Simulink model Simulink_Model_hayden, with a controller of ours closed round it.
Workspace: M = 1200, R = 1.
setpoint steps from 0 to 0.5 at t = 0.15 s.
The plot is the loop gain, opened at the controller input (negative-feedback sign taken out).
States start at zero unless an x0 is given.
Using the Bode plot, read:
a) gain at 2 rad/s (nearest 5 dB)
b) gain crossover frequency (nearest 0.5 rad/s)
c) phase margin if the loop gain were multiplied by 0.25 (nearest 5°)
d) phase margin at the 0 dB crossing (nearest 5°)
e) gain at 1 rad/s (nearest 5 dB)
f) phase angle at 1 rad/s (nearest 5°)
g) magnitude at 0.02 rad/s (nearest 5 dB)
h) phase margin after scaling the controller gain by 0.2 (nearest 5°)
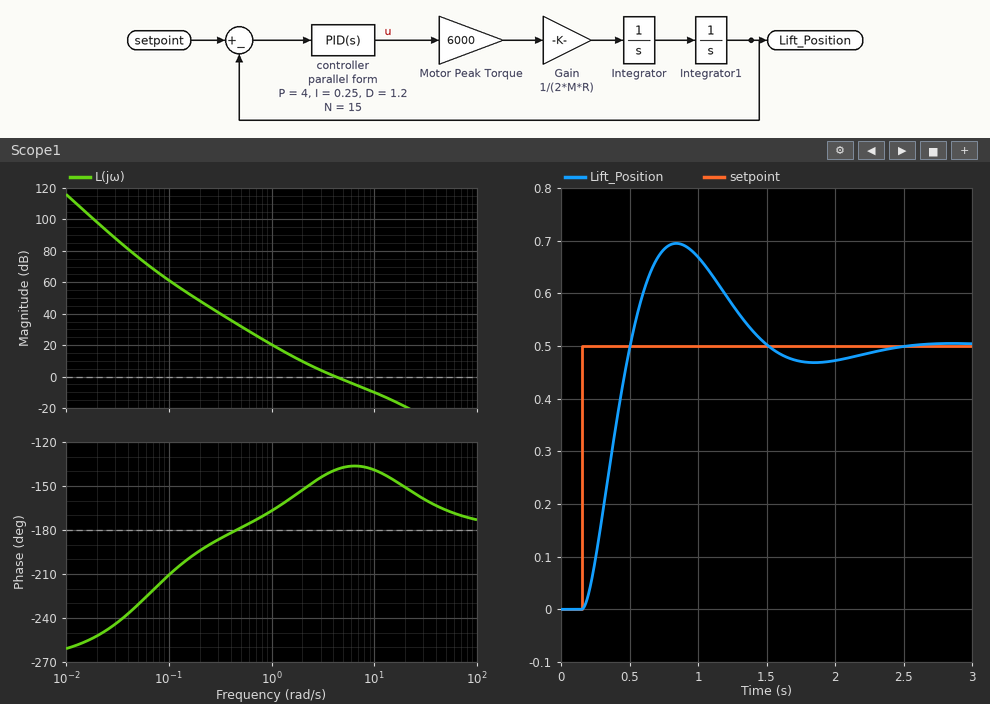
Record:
10 dB
4.0 rad/s
25°
40°
20 dB
-165°
100 dB
20°
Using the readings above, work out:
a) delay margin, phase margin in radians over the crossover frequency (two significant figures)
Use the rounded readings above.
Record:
0.17 s
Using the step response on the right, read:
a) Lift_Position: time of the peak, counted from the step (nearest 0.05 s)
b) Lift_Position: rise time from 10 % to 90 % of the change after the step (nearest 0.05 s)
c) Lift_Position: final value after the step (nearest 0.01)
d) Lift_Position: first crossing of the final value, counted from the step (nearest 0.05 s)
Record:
0.70 s
0.25 s
0.50
0.35 s
